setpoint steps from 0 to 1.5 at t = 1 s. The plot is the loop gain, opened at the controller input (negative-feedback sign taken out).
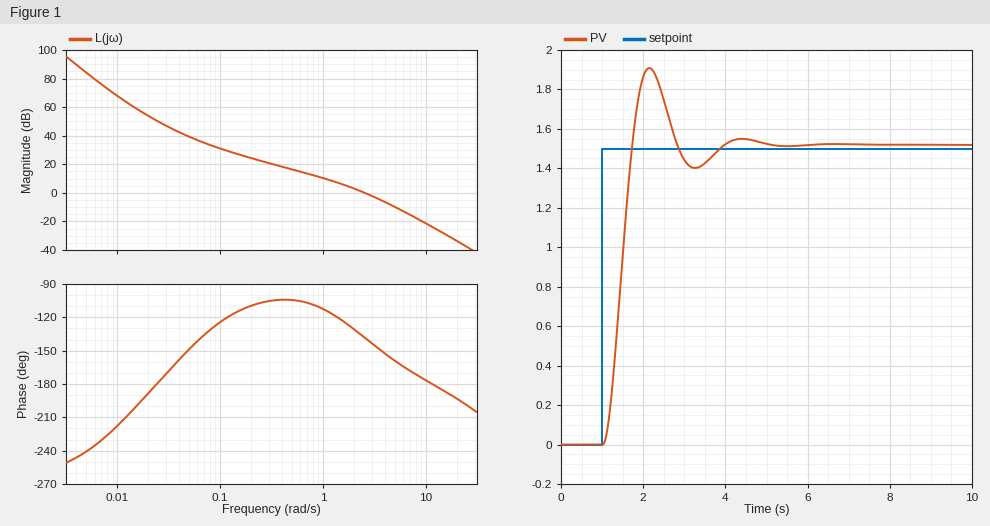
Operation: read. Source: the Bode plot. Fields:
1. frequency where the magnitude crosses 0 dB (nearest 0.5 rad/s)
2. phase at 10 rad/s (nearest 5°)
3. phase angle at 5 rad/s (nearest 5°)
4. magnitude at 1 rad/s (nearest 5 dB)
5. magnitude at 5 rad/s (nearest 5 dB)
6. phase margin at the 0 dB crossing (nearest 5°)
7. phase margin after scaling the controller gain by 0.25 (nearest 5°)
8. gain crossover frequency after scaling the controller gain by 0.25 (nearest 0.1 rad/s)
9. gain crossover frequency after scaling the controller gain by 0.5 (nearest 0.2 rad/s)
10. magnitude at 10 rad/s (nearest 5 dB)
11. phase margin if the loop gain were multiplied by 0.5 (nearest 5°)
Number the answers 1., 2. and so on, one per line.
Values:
1. 2.5 rad/s
2. -175°
3. -160°
4. 10 dB
5. -10 dB
6. 40°
7. 70°
8. 0.8 rad/s
9. 1.6 rad/s
10. -20 dB
11. 55°
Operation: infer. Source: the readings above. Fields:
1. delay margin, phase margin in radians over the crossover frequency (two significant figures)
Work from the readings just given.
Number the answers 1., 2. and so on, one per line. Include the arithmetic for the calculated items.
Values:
1. 40 × π / 180 / 2.5 = 0.28 s
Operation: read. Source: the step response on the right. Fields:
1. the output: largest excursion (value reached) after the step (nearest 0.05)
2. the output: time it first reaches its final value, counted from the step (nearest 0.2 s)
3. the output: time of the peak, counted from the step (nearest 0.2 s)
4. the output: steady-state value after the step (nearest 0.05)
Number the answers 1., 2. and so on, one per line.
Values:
1. 1.90
2. 0.8 s
3. 1.2 s
4. 1.50
